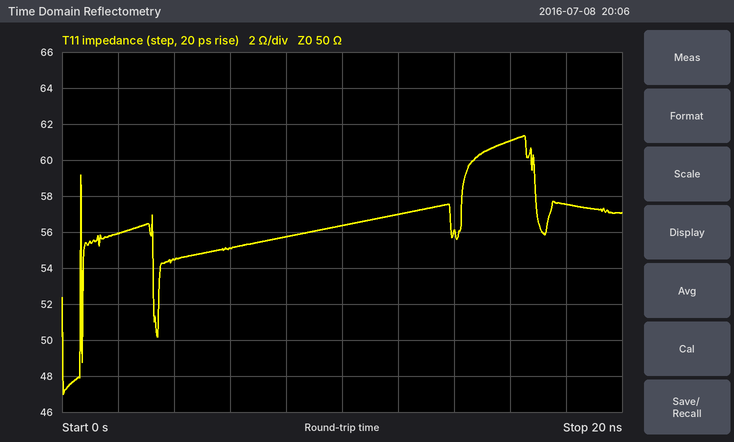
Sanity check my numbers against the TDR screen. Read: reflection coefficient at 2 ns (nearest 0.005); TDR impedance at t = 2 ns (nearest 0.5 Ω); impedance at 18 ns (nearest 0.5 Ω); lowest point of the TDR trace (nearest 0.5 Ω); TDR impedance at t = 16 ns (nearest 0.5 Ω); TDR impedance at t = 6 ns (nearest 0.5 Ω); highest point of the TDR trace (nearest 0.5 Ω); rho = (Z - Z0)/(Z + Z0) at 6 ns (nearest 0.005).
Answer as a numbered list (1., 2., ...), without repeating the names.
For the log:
1. +0.055
2. 56.0 Ω
3. 57.5 Ω
4. 47.0 Ω
5. 61.0 Ω
6. 55.0 Ω
7. 61.5 Ω
8. +0.050
